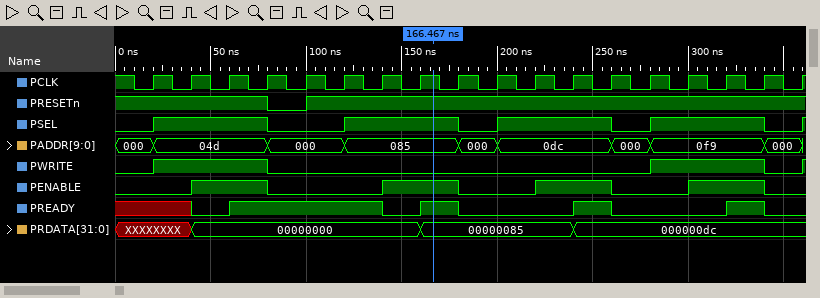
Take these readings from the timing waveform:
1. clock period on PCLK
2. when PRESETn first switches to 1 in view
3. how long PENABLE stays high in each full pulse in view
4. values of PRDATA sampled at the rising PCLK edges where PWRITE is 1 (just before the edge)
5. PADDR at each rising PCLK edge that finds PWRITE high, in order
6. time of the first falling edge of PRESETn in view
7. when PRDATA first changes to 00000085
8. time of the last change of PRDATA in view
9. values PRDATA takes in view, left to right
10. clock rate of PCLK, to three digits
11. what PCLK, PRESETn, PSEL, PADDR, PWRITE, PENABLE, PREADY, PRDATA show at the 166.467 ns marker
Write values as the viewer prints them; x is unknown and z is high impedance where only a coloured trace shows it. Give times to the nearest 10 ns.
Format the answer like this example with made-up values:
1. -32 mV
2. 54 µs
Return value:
1. 20 ns
2. 100 ns
3. 40 ns, 40 ns, 40 ns, 40 ns
4. XXXXXXXX, 00000000, 00000000, 000000dc, 000000dc, 000000dc
5. 04d, 04d, 04d, 0f9, 0f9, 0f9
6. 80 ns
7. 160 ns
8. 240 ns
9. XXXXXXXX, 00000000, 00000085, 000000dc
10. 50.0 MHz
11. PCLK=1, PRESETn=1, PSEL=1, PADDR=085, PWRITE=0, PENABLE=1, PREADY=1, PRDATA=00000085
